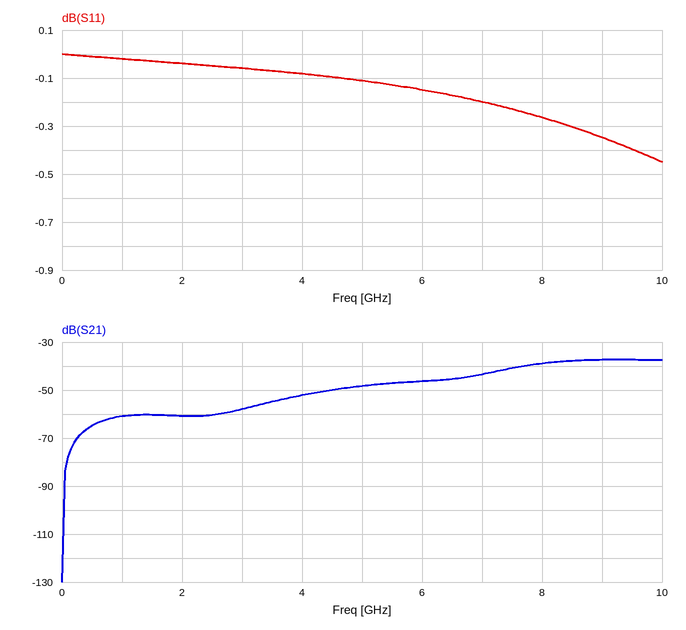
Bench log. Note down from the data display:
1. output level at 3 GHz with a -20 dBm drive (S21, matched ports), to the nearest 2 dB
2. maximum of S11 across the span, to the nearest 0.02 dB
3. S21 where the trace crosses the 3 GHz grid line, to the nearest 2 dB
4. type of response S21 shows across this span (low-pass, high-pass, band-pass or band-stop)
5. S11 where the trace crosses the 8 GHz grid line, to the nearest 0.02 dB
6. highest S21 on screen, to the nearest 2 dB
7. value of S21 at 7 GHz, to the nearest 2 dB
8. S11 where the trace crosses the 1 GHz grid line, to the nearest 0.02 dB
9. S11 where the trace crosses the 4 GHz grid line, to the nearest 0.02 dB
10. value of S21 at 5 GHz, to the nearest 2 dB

-78 dBm
0.00 dB
-58 dB
high-pass
-0.26 dB
-38 dB
-44 dB
-0.02 dB
-0.08 dB
-48 dB
